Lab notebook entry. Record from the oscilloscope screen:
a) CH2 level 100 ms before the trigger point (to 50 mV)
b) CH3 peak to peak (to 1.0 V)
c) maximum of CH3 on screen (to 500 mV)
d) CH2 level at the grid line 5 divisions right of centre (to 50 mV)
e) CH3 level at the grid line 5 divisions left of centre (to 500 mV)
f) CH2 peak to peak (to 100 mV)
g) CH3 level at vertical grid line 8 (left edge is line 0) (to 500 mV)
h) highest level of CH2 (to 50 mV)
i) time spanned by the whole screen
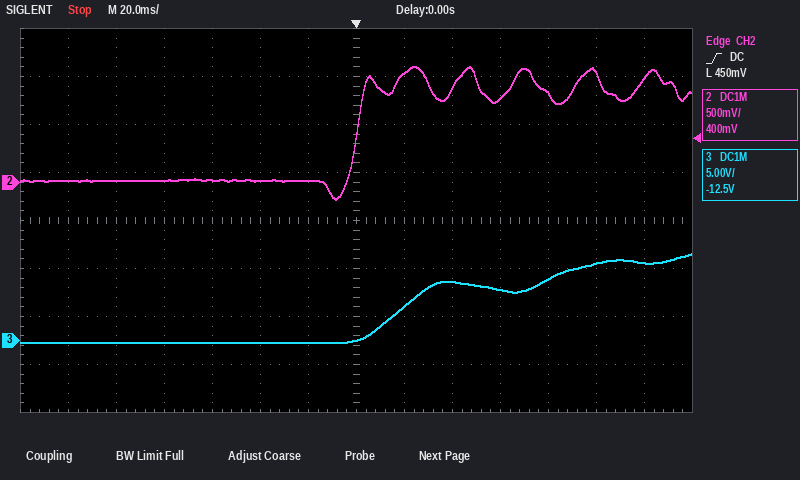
0 mV
9.0 V
9.0 V
1.15 V
0.0 V
1.40 V
3.5 V
1.20 V
280 ms
